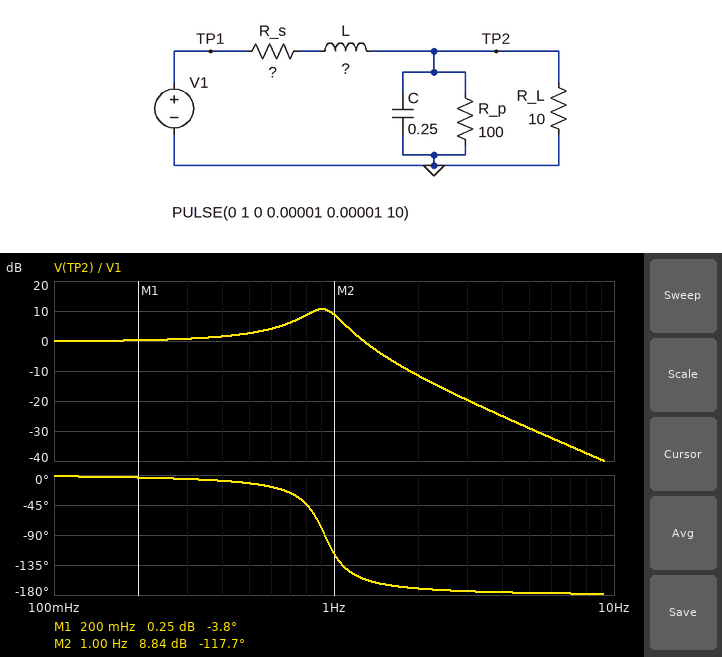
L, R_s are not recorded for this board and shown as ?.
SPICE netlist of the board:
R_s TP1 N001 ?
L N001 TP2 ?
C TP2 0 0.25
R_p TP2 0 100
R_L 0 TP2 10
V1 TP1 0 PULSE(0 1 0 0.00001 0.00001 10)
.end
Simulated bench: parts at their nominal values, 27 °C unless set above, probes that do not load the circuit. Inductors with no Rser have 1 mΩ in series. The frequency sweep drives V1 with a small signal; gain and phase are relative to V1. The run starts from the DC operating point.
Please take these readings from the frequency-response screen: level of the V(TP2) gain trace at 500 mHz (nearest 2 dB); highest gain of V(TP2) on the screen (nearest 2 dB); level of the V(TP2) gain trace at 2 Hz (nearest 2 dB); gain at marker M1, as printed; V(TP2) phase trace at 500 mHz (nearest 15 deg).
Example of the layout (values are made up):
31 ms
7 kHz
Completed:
2 dB
10 dB
-12 dB
0.25 dB
-15 deg
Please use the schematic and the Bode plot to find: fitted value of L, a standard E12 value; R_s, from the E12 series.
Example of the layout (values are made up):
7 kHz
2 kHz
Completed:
120 mH
0.15 Ω
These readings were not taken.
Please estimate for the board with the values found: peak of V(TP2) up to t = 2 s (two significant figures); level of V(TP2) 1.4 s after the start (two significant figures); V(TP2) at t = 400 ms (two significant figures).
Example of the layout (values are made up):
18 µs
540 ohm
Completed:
1.6 V
1.0 V
1.4 V
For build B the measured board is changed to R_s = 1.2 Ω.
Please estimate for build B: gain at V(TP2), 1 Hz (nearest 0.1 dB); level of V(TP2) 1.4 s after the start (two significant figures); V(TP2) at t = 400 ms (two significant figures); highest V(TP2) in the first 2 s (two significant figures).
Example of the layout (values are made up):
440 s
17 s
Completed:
-5.9 dB
880 mV
680 mV
890 mV
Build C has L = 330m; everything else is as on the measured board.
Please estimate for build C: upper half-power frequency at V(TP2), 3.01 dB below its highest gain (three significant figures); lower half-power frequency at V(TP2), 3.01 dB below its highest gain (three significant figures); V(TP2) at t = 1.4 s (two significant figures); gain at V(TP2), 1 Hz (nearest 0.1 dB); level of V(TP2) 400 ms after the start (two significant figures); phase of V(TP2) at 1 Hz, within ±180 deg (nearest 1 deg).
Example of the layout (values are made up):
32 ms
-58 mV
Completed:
617 mHz
472 mHz
970 mV
-7.2 dB
730 mV
-168 deg
